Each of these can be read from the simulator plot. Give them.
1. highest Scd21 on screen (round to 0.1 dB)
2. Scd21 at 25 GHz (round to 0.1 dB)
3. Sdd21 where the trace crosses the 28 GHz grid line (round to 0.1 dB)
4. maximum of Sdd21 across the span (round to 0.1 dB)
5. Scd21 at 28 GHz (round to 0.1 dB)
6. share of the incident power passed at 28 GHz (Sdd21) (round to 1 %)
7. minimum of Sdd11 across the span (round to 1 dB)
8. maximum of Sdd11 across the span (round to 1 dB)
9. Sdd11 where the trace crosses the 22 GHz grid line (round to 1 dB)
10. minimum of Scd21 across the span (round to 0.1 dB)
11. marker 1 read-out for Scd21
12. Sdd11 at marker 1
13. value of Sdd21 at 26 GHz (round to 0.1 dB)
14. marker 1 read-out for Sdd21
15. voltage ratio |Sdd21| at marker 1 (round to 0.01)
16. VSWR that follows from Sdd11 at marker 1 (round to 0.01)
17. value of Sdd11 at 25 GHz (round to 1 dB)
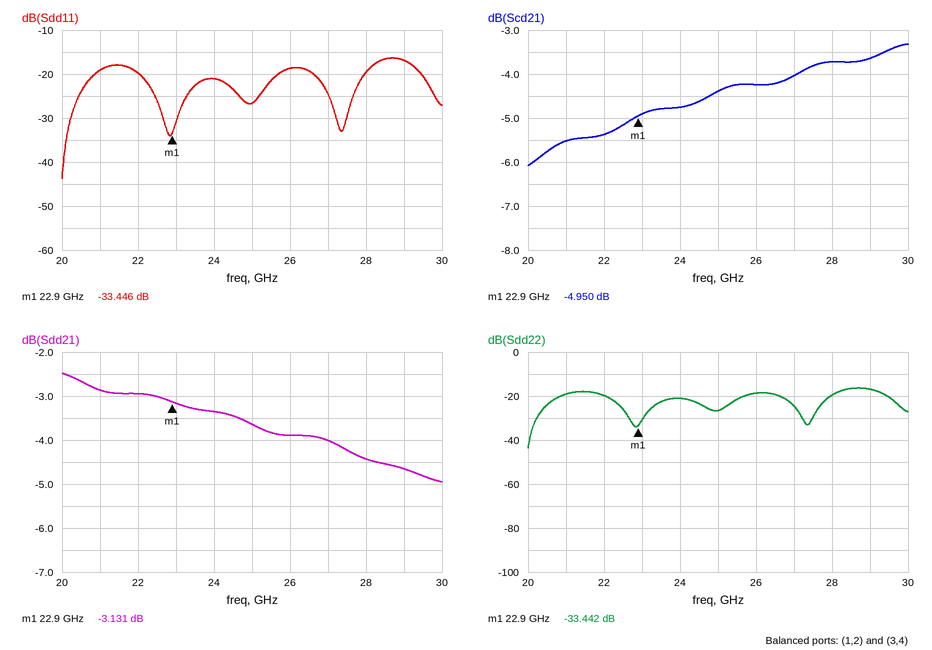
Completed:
-3.3 dB
-4.4 dB
-4.4 dB
-2.5 dB
-3.7 dB
36 %
-44 dB
-16 dB
-20 dB
-6.1 dB
-4.950 dB
-33.446 dB
-3.9 dB
-3.131 dB
0.70
1.04
-27 dB
